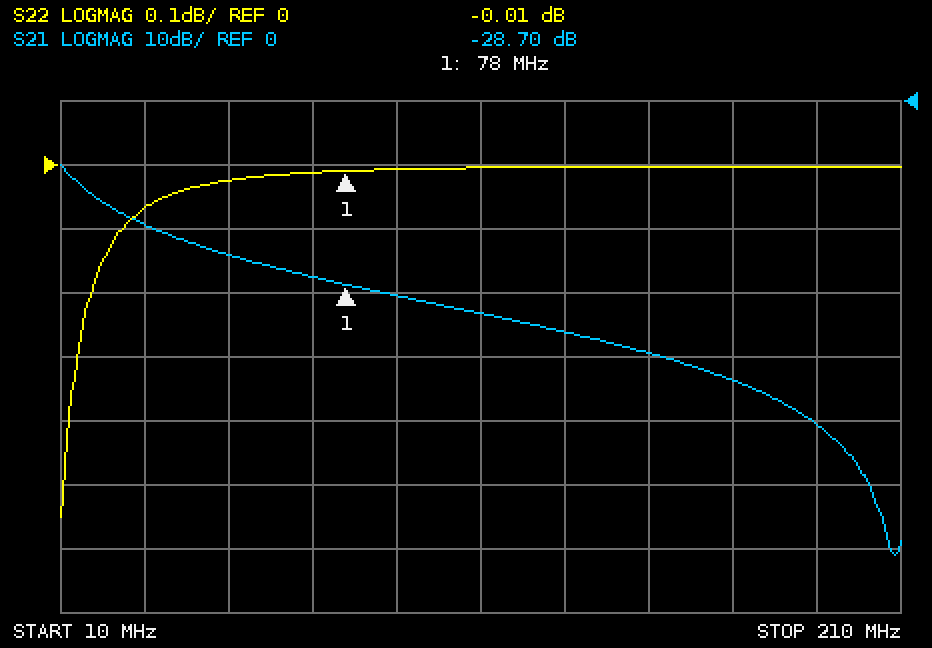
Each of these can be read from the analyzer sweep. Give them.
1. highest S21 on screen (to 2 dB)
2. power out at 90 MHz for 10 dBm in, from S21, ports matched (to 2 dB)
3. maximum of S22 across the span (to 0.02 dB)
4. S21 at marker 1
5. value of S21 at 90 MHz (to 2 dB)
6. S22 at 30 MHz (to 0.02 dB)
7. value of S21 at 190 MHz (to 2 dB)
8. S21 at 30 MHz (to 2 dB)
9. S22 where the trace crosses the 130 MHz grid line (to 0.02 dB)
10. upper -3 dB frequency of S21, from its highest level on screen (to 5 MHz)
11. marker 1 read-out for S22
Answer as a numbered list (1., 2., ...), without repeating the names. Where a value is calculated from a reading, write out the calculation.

1. -10 dB
2. 10 dBm + (-30 dB) = -20 dBm
3. 0.00 dB
4. -28.70 dB
5. -30 dB
6. -0.06 dB
7. -50 dB
8. -20 dB
9. 0.00 dB
10. 15 MHz
11. -0.01 dB
